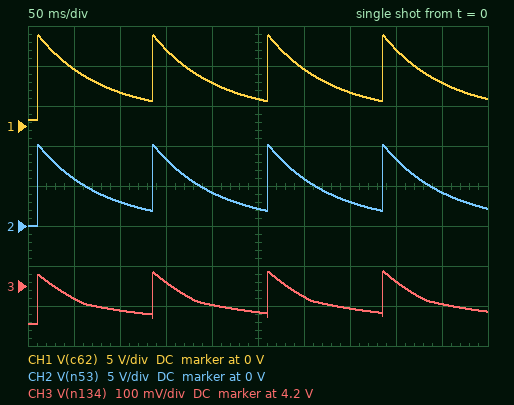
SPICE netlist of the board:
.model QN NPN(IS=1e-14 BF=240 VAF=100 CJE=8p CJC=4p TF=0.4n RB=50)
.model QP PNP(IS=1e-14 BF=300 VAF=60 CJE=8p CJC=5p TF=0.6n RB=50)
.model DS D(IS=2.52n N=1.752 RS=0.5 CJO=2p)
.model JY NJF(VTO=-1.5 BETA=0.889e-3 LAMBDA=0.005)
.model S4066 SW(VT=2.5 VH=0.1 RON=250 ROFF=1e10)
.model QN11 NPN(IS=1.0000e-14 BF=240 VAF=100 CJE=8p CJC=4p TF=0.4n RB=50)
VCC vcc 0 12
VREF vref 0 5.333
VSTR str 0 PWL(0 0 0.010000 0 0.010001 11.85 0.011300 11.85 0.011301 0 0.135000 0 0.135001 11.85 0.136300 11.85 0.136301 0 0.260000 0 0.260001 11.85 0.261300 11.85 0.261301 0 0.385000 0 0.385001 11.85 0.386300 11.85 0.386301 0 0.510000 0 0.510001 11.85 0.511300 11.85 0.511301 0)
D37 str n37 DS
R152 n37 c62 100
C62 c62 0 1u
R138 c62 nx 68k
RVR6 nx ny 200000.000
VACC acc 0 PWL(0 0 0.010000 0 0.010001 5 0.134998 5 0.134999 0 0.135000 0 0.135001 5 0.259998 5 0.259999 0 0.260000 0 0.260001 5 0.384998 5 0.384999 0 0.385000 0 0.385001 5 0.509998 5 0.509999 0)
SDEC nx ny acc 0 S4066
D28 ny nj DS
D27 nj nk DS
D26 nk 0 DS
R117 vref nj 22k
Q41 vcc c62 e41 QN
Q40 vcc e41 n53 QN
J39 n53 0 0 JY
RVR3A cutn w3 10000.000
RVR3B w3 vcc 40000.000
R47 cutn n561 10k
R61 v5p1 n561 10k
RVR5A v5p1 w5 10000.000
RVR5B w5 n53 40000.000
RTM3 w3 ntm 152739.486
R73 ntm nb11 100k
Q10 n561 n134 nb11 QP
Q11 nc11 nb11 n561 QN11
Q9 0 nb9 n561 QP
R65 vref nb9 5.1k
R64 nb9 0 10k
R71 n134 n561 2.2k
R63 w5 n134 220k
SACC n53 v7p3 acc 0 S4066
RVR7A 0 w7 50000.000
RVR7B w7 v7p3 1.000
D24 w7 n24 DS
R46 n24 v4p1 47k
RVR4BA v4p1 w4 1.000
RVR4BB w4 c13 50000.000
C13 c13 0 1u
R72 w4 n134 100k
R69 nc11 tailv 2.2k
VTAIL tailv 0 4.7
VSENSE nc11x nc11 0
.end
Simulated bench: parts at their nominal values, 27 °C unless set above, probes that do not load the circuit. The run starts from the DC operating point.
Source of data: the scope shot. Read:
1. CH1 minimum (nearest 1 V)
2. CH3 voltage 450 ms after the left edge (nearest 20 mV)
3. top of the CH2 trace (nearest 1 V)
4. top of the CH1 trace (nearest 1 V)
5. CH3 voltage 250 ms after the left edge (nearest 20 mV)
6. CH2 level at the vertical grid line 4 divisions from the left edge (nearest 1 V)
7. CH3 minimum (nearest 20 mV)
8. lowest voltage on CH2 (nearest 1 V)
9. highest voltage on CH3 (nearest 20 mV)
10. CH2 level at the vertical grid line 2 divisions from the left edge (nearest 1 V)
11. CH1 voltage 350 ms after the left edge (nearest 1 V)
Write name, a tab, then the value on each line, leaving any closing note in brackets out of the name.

CH1 minimum	1 V
CH3 voltage 450 ms after the left edge	4.16 V
top of the CH2 trace	10 V
top of the CH1 trace	11 V
CH3 voltage 250 ms after the left edge	4.14 V
CH2 level at the vertical grid line 4 divisions from the left edge	4 V
CH3 minimum	4.10 V
lowest voltage on CH2	0 V
highest voltage on CH3	4.24 V
CH2 level at the vertical grid line 2 divisions from the left edge	3 V
CH1 voltage 350 ms after the left edge	4 V
